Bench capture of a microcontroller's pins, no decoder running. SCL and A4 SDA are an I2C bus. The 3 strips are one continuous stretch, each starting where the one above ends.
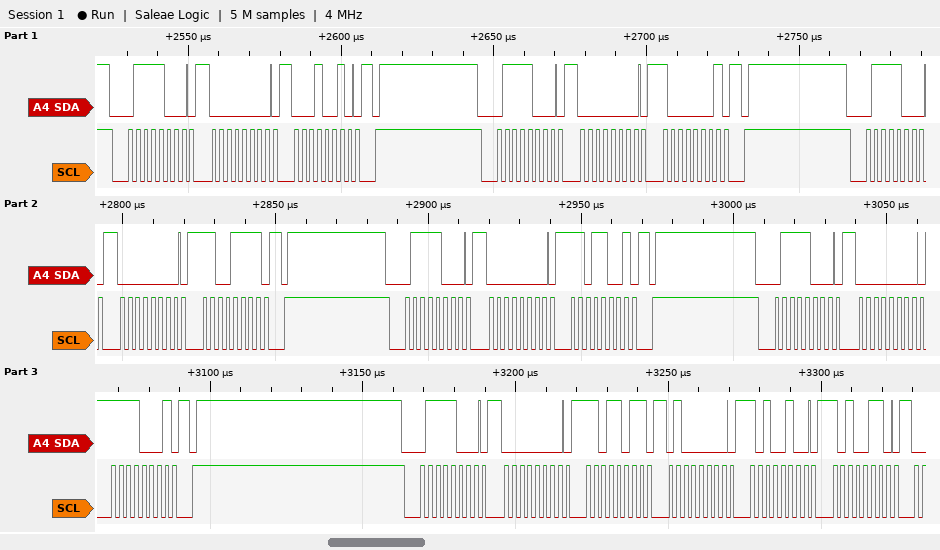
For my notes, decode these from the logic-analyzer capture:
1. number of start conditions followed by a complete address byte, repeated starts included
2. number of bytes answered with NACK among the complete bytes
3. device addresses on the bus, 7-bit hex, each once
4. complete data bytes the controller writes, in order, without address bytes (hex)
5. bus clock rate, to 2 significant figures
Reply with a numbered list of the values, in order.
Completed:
1. 6
2. 0
3. 0x3C
4. 00 12 00 81 00 CF 00 D9 00 F1 00 DB 40 A4 A6
5. 400 kHz
